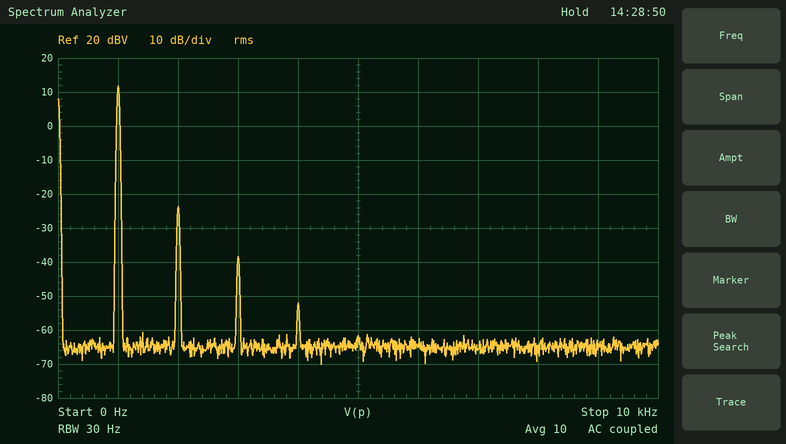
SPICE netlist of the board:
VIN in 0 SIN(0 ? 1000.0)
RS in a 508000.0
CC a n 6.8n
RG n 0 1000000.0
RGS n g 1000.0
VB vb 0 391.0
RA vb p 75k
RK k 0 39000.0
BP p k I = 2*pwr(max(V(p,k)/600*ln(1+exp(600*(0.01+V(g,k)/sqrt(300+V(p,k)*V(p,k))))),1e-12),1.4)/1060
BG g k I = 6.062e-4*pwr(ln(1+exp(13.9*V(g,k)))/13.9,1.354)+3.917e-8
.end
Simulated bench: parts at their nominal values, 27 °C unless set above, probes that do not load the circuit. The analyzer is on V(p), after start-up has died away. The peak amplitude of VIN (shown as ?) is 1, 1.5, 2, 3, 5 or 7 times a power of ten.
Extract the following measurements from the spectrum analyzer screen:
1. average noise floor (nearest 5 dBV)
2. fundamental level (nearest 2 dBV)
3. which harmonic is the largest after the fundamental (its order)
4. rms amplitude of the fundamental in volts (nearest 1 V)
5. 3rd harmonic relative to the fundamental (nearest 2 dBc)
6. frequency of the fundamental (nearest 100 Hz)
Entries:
-65 dBV
12 dBV
2
4 V
-50 dBc
1.0 kHz
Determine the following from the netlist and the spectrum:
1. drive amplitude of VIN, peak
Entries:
5 V
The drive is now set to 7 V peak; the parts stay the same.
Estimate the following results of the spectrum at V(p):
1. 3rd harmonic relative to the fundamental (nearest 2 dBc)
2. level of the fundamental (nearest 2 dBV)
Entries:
-42 dBc
14 dBV
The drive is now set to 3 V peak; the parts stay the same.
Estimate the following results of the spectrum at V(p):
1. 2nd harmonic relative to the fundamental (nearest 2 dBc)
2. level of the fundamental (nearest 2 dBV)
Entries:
-40 dBc
8 dBV
